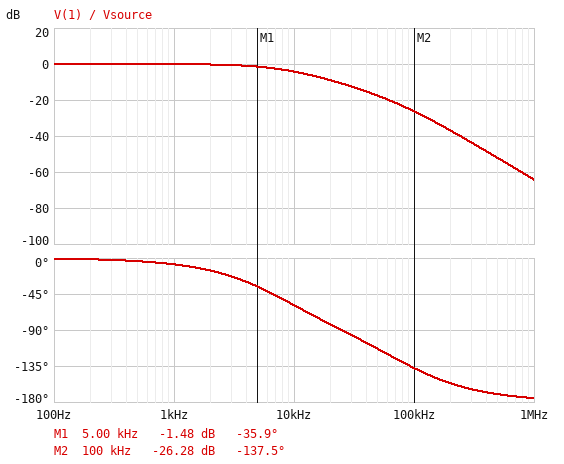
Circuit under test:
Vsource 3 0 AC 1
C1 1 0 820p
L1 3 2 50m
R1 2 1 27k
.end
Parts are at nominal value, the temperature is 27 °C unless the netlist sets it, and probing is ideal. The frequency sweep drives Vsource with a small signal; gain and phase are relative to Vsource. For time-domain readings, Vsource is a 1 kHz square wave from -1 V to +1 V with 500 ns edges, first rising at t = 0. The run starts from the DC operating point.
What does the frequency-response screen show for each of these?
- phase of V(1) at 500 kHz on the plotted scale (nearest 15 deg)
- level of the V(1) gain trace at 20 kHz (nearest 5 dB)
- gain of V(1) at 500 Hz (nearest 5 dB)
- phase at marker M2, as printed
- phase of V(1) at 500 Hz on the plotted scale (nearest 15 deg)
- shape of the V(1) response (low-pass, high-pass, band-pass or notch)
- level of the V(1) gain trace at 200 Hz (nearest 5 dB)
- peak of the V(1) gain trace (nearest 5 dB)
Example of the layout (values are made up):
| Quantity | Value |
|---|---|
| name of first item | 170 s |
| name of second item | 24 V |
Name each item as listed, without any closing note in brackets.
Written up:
| Quantity | Value |
|---|---|
| phase of V(1) at 500 kHz on the plotted scale | -165 deg |
| level of the V(1) gain trace at 20 kHz | -10 dB |
| gain of V(1) at 500 Hz | 0 dB |
| phase at marker M2, as printed | -137.5 deg |
| phase of V(1) at 500 Hz on the plotted scale | 0 deg |
| shape of the V(1) response | low-pass |
| level of the V(1) gain trace at 200 Hz | 0 dB |
| peak of the V(1) gain trace | 0 dB |
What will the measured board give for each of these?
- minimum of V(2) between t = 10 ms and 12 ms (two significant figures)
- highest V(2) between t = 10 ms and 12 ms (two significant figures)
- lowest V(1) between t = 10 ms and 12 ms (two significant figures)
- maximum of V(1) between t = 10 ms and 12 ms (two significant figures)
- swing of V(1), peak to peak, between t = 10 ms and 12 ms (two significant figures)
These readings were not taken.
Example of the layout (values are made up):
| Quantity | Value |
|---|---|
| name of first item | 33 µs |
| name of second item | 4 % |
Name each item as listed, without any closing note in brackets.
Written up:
| Quantity | Value |
|---|---|
| minimum of V(2) between t = 10 ms and 12 ms | -1.1 V |
| highest V(2) between t = 10 ms and 12 ms | 1.1 V |
| lowest V(1) between t = 10 ms and 12 ms | -1.0 V |
| maximum of V(1) between t = 10 ms and 12 ms | 1.0 V |
| swing of V(1), peak to peak, between t = 10 ms and 12 ms | 2.0 V |
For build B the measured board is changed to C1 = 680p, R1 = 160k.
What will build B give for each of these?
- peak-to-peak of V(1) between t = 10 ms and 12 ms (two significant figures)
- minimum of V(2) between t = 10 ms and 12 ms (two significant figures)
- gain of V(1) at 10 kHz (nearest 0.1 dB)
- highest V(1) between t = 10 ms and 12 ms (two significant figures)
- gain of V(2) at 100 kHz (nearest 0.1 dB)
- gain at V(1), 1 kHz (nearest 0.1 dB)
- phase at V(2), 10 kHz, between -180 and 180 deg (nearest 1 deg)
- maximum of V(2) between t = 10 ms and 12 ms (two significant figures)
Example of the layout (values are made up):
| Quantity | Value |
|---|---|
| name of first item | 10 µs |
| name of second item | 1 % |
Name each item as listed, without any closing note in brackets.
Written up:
| Quantity | Value |
|---|---|
| peak-to-peak of V(1) between t = 10 ms and 12 ms | 2.0 V |
| minimum of V(2) between t = 10 ms and 12 ms | -1.0 V |
| gain of V(1) at 10 kHz | -16.8 dB |
| highest V(1) between t = 10 ms and 12 ms | 980 mV |
| gain of V(2) at 100 kHz | -0.1 dB |
| gain at V(1), 1 kHz | -1.7 dB |
| phase at V(2), 10 kHz, between -180 and 180 deg | -1 deg |
| maximum of V(2) between t = 10 ms and 12 ms | 1.0 V |
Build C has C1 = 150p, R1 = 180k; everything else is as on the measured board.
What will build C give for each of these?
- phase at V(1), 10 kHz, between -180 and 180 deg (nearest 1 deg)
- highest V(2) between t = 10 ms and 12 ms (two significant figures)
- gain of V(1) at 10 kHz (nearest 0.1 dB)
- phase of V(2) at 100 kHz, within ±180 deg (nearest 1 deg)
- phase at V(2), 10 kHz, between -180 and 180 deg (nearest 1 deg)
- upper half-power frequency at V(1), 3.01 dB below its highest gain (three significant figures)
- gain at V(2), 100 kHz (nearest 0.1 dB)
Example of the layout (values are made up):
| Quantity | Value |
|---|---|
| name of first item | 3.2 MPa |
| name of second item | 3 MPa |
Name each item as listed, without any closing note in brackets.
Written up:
| Quantity | Value |
|---|---|
| phase at V(1), 10 kHz, between -180 and 180 deg | -60 deg |
| highest V(2) between t = 10 ms and 12 ms | 1.0 V |
| gain of V(1) at 10 kHz | -5.8 dB |
| phase of V(2) at 100 kHz, within ±180 deg | -10 deg |
| phase at V(2), 10 kHz, between -180 and 180 deg | -1 deg |
| upper half-power frequency at V(1), 3.01 dB below its highest gain | 5.96 kHz |
| gain at V(2), 100 kHz | 0 dB |
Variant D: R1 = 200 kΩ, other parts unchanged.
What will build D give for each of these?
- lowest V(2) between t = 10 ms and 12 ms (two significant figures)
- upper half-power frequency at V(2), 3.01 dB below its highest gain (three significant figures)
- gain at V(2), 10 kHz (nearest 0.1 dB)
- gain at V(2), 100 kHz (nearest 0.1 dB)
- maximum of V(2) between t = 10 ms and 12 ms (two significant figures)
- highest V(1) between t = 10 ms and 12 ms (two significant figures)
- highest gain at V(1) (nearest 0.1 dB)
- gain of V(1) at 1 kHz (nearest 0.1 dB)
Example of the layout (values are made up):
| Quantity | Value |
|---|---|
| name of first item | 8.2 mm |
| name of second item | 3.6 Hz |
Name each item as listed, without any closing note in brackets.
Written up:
| Quantity | Value |
|---|---|
| lowest V(2) between t = 10 ms and 12 ms | -1.0 V |
| upper half-power frequency at V(2), 3.01 dB below its highest gain | 636 kHz |
| gain at V(2), 10 kHz | 0 dB |
| gain at V(2), 100 kHz | -0.1 dB |
| maximum of V(2) between t = 10 ms and 12 ms | 1.0 V |
| highest V(1) between t = 10 ms and 12 ms | 910 mV |
| highest gain at V(1) | 0 dB |
| gain of V(1) at 1 kHz | -3.1 dB |
